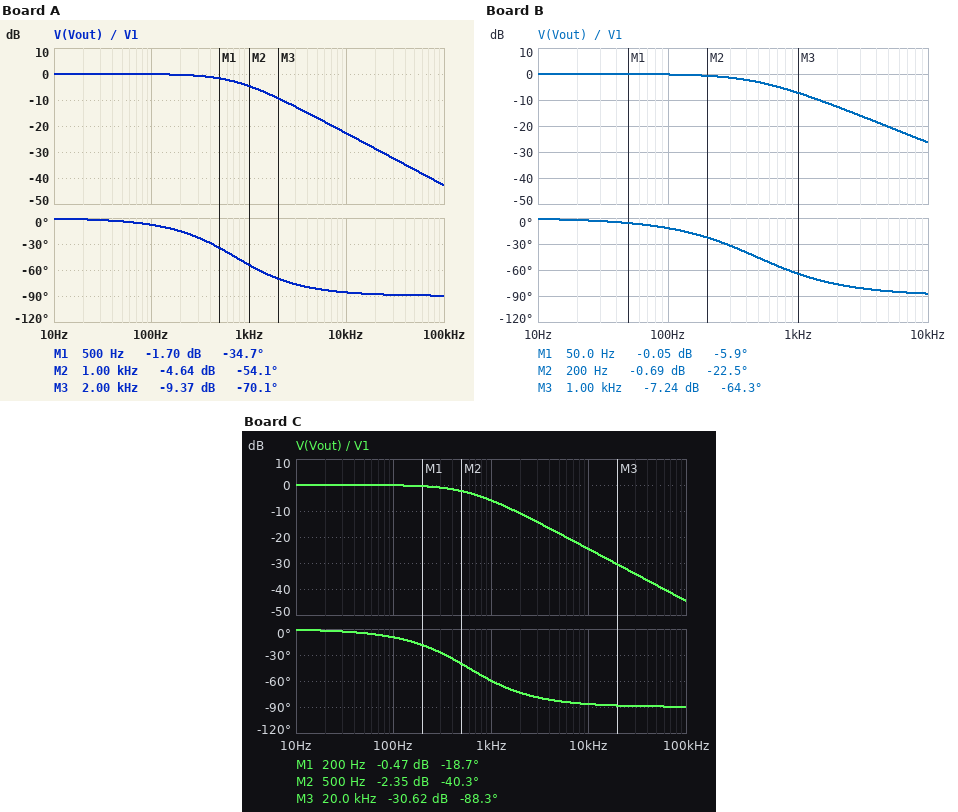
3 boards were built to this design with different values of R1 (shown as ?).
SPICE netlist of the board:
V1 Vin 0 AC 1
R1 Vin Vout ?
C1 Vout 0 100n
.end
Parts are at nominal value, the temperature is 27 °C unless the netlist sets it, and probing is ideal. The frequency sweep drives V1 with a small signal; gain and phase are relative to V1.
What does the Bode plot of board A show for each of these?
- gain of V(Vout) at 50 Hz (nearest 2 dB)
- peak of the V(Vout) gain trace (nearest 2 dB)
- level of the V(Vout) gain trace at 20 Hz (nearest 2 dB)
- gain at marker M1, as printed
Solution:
0 dB
0 dB
0 dB
-1.70 dB
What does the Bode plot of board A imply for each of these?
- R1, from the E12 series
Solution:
2.2 kΩ
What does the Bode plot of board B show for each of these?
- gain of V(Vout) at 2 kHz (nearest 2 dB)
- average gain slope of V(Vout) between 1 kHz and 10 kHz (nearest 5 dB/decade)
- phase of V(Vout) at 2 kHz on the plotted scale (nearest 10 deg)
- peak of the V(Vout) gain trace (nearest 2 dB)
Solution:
-12 dB
-20 dB/decade
-80 deg
0 dB
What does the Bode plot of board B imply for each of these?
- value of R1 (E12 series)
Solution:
3.3 kΩ
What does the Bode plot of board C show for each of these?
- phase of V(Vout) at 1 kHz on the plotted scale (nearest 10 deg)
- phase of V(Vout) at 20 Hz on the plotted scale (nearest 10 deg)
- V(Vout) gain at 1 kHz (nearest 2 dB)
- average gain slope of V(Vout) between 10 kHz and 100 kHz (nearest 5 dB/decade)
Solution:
-60 deg
0 deg
-6 dB
-20 dB/decade
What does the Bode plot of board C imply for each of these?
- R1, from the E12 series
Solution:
2.7 kΩ
